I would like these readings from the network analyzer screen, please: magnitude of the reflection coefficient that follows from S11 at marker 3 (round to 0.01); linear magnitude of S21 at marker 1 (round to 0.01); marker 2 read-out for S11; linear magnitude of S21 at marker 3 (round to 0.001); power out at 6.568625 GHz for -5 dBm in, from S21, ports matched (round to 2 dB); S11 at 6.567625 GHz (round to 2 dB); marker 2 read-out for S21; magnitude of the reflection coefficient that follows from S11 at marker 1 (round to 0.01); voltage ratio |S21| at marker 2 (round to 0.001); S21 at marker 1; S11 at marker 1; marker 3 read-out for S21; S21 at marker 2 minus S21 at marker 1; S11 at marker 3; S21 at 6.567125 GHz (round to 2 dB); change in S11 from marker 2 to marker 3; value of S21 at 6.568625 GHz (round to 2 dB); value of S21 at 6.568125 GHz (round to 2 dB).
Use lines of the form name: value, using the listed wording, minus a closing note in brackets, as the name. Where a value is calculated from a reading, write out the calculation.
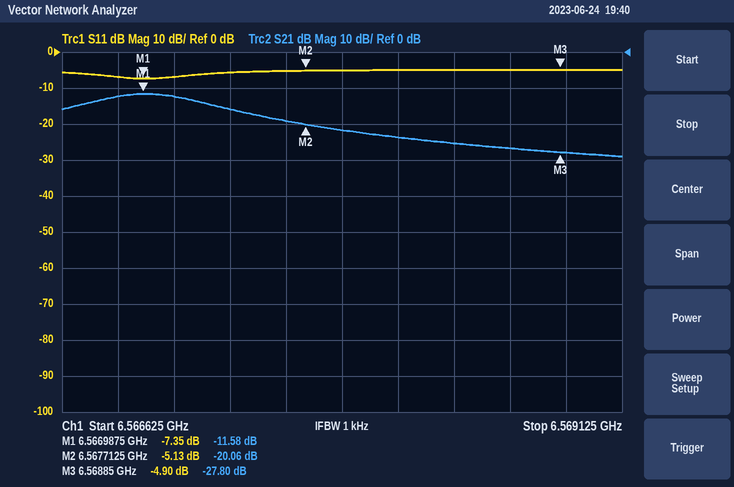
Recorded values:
magnitude of the reflection coefficient that follows from S11 at marker 3: 10^(-4.9/20) ≈ 0.57
linear magnitude of S21 at marker 1: 10^(-11.58/20) ≈ 0.26
marker 2 read-out for S11: -5.13 dB
linear magnitude of S21 at marker 3: 10^(-27.8/20) ≈ 0.041
power out at 6.568625 GHz for -5 dBm in, from S21, ports matched: -5 dBm + (-26 dB) = -32 dBm
S11 at 6.567625 GHz: -6 dB
marker 2 read-out for S21: -20.06 dB
magnitude of the reflection coefficient that follows from S11 at marker 1: 10^(-7.35/20) ≈ 0.43
voltage ratio |S21| at marker 2: 10^(-20.06/20) ≈ 0.099
S21 at marker 1: -11.58 dB
S11 at marker 1: -7.35 dB
marker 3 read-out for S21: -27.80 dB
S21 at marker 2 minus S21 at marker 1: -20.06 − (-11.58) = -8.48 dB
S11 at marker 3: -4.90 dB
S21 at 6.567125 GHz: -12 dB
change in S11 from marker 2 to marker 3: -4.9 − (-5.13) = 0.23 dB
value of S21 at 6.568625 GHz: -26 dB
value of S21 at 6.568125 GHz: -24 dB
